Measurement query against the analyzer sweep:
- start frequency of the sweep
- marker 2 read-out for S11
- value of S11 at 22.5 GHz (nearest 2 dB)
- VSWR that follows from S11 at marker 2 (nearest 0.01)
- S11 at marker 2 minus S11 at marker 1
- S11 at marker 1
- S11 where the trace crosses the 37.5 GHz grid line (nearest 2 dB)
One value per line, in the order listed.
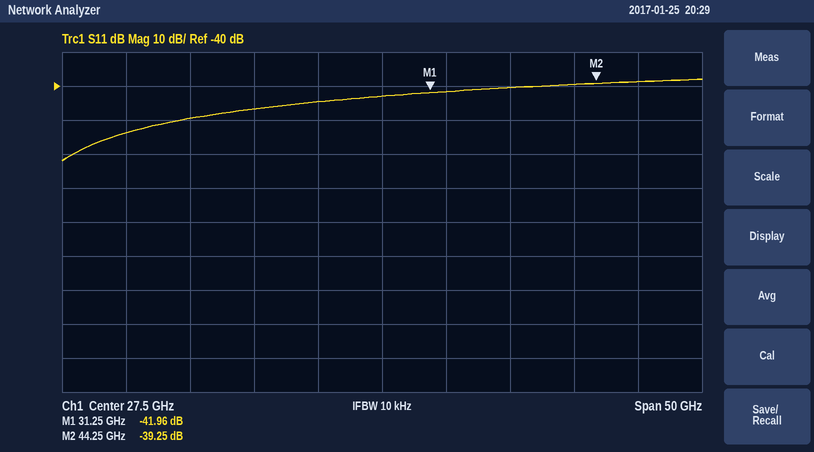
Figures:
2.5 GHz
-39.25 dB
-44 dB
1.02
2.71 dB
-41.96 dB
-40 dB
